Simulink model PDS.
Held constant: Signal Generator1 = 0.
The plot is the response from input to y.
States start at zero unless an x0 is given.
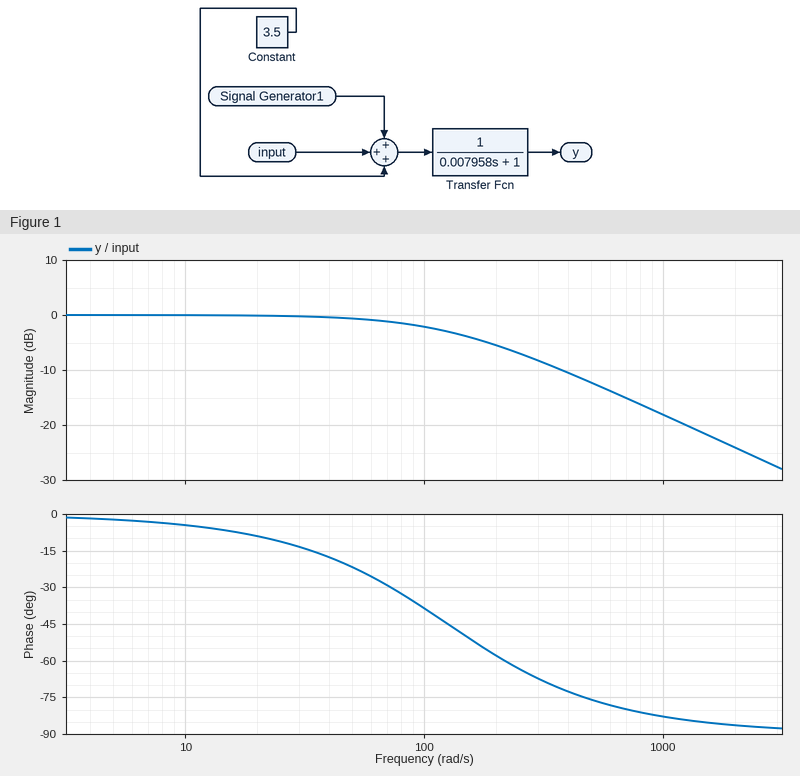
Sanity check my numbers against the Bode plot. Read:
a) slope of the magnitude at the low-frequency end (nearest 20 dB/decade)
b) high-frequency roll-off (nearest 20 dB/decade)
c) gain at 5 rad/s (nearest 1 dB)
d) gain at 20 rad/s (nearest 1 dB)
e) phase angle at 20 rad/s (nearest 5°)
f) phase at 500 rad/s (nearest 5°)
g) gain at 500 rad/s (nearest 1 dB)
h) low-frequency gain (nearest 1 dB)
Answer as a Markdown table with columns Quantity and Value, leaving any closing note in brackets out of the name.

| Quantity | Value |
|---|---|
| slope of the magnitude at the low-frequency end | 0 dB/decade |
| high-frequency roll-off | -20 dB/decade |
| gain at 5 rad/s | 0 dB |
| gain at 20 rad/s | 0 dB |
| phase angle at 20 rad/s | -10° |
| phase at 500 rad/s | -75° |
| gain at 500 rad/s | -12 dB |
| low-frequency gain | 0 dB |
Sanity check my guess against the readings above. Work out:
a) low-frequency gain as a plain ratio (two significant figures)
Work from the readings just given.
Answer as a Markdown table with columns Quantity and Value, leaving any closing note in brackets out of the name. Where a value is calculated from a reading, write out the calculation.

| Quantity | Value |
|---|---|
| low-frequency gain as a plain ratio | 10^(0 / 20) = 1.0 |
